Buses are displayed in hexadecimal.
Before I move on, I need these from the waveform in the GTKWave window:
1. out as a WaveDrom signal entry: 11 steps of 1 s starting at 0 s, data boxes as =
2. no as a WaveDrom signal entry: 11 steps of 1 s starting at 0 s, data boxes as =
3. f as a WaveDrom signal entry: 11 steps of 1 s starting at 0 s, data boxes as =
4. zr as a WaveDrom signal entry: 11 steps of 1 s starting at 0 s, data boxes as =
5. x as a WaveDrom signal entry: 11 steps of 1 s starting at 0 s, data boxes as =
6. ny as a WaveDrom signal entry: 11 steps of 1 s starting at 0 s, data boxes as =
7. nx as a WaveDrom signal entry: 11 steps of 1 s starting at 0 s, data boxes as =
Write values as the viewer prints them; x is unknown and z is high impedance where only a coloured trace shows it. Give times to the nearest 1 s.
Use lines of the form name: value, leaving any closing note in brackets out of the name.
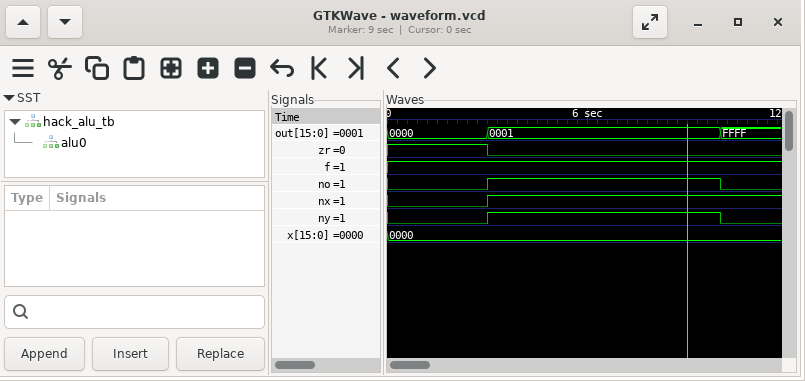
out as a WaveDrom signal entry: 11 steps of 1 s starting at 0 s, data boxes as =: {name: 'out', wave: '=..=......=', data: '0000 0001 FFFF'}
no as a WaveDrom signal entry: 11 steps of 1 s starting at 0 s, data boxes as =: {name: 'no', wave: '0..1......0'}
f as a WaveDrom signal entry: 11 steps of 1 s starting at 0 s, data boxes as =: {name: 'f', wave: '1..........'}
zr as a WaveDrom signal entry: 11 steps of 1 s starting at 0 s, data boxes as =: {name: 'zr', wave: '1..0.......'}
x as a WaveDrom signal entry: 11 steps of 1 s starting at 0 s, data boxes as =: {name: 'x', wave: '=..........', data: '0000'}
ny as a WaveDrom signal entry: 11 steps of 1 s starting at 0 s, data boxes as =: {name: 'ny', wave: '0..1......0'}
nx as a WaveDrom signal entry: 11 steps of 1 s starting at 0 s, data boxes as =: {name: 'nx', wave: '0..1.......'}
